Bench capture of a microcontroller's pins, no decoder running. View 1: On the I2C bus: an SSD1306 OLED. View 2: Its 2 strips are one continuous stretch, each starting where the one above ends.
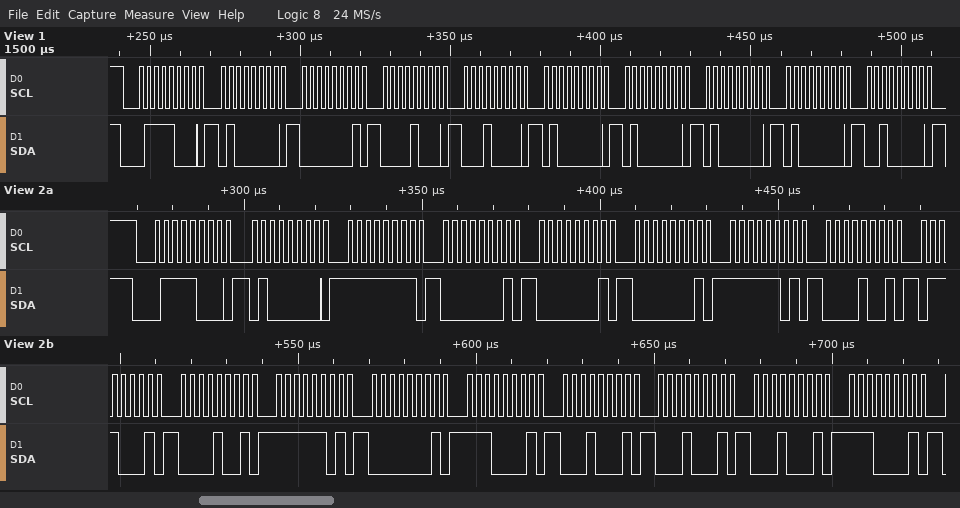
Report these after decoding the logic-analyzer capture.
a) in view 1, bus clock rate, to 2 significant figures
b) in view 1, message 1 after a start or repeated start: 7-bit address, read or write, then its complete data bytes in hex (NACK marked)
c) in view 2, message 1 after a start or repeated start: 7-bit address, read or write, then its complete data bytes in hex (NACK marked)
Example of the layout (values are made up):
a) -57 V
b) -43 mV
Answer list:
a) 400 kHz
b) 0x3C write: 40 01 08 10 40 40 40 40 20
c) 0x3C write: 40 FF 01 01 01 FD 09 71 09 FD 01 E1 11 11 11 E1
